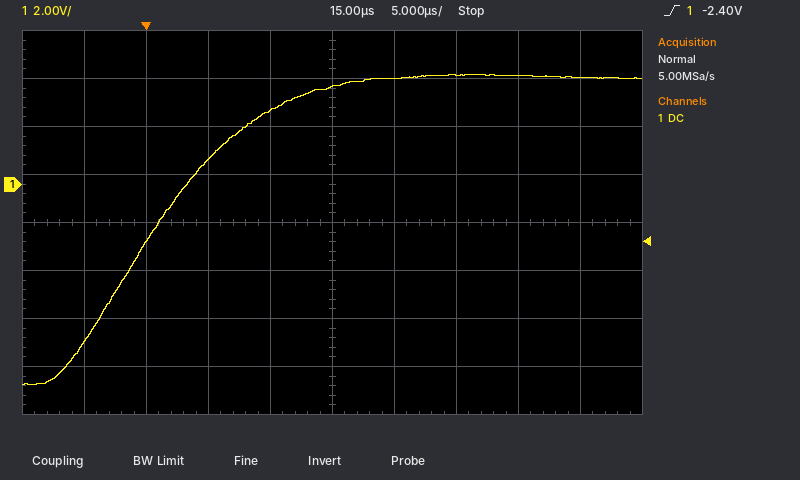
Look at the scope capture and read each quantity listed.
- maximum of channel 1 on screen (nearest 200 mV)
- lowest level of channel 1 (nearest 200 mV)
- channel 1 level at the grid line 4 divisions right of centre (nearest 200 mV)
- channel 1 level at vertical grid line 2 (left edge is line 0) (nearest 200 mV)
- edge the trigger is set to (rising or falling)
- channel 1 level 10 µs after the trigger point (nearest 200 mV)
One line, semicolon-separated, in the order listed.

4.6 V; -8.4 V; 4.4 V; -2.4 V; rising; 3.0 V
